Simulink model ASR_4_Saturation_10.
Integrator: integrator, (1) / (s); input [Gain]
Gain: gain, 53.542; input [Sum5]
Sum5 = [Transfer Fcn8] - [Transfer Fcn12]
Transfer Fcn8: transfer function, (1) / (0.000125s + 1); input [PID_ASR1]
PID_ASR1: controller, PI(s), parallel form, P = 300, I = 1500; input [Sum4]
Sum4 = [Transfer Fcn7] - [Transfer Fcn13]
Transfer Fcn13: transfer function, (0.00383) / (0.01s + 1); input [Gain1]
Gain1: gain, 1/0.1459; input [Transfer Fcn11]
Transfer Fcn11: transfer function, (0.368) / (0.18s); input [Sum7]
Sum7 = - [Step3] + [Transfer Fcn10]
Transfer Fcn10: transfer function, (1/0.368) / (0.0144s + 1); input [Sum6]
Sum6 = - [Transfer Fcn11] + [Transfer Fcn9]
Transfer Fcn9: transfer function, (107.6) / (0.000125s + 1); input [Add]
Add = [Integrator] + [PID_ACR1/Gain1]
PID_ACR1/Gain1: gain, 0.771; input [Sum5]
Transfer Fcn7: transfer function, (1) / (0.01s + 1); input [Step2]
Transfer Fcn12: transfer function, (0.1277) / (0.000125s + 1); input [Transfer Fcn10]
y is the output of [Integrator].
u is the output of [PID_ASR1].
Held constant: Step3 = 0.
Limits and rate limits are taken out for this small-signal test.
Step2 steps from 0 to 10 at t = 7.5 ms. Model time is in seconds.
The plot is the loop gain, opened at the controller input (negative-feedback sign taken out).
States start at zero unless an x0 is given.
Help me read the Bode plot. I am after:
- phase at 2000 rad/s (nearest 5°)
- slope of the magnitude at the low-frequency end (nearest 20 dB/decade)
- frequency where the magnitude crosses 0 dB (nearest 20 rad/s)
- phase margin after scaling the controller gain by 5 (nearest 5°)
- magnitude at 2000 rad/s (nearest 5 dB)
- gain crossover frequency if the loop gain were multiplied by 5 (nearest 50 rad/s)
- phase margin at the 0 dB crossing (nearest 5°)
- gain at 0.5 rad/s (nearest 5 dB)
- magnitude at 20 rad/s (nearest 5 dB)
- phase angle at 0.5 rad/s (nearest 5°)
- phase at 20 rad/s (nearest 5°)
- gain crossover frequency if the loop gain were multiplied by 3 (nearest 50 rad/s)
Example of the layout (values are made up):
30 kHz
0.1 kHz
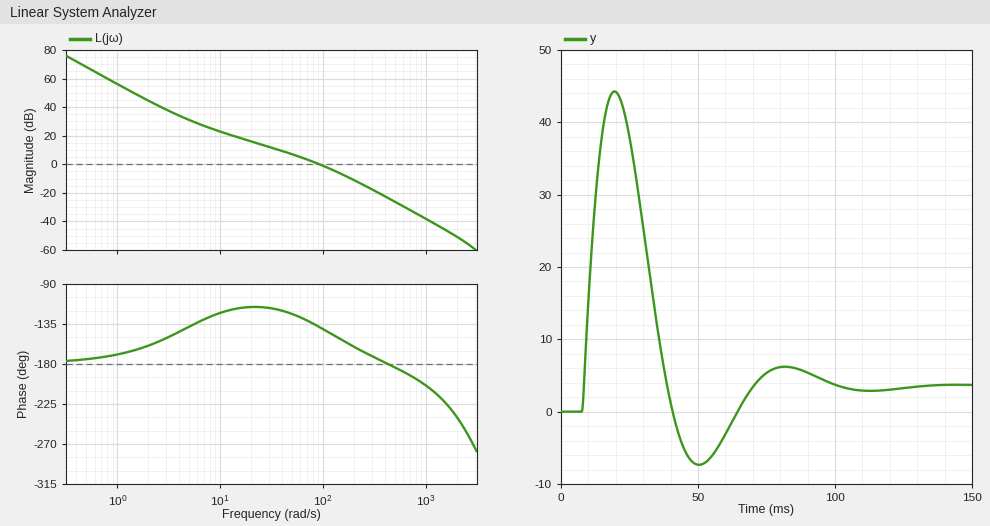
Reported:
-240°
-40 dB/decade
100 rad/s
15°
-50 dB
250 rad/s
40°
70 dB
15 dB
-175°
-115°
200 rad/s
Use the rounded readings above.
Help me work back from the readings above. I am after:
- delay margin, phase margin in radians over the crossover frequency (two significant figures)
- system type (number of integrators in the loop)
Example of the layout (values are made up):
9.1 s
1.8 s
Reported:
0.0070 s
2
